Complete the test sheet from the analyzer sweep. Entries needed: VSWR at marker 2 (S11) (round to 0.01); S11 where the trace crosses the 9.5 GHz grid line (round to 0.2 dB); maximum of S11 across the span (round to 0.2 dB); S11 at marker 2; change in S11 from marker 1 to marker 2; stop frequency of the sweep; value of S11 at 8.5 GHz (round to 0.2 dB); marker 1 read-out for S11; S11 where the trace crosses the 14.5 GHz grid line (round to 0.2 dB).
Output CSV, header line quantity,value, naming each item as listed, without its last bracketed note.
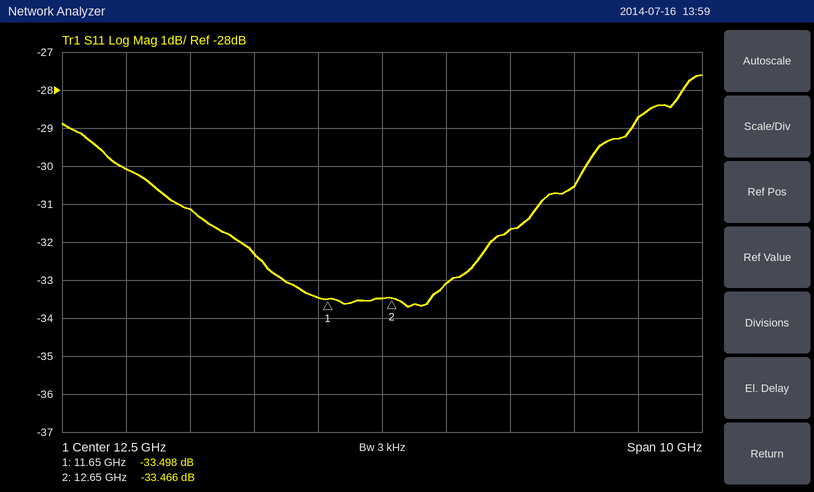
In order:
quantity,value
VSWR at marker 2 (S11),1.04
S11 where the trace crosses the 9.5 GHz grid line,-31.2 dB
maximum of S11 across the span,-27.6 dB
S11 at marker 2,-33.466 dB
change in S11 from marker 1 to marker 2,0.032 dB
stop frequency of the sweep,17.5 GHz
value of S11 at 8.5 GHz,-30.0 dB
marker 1 read-out for S11,-33.498 dB
S11 where the trace crosses the 14.5 GHz grid line,-31.6 dB
